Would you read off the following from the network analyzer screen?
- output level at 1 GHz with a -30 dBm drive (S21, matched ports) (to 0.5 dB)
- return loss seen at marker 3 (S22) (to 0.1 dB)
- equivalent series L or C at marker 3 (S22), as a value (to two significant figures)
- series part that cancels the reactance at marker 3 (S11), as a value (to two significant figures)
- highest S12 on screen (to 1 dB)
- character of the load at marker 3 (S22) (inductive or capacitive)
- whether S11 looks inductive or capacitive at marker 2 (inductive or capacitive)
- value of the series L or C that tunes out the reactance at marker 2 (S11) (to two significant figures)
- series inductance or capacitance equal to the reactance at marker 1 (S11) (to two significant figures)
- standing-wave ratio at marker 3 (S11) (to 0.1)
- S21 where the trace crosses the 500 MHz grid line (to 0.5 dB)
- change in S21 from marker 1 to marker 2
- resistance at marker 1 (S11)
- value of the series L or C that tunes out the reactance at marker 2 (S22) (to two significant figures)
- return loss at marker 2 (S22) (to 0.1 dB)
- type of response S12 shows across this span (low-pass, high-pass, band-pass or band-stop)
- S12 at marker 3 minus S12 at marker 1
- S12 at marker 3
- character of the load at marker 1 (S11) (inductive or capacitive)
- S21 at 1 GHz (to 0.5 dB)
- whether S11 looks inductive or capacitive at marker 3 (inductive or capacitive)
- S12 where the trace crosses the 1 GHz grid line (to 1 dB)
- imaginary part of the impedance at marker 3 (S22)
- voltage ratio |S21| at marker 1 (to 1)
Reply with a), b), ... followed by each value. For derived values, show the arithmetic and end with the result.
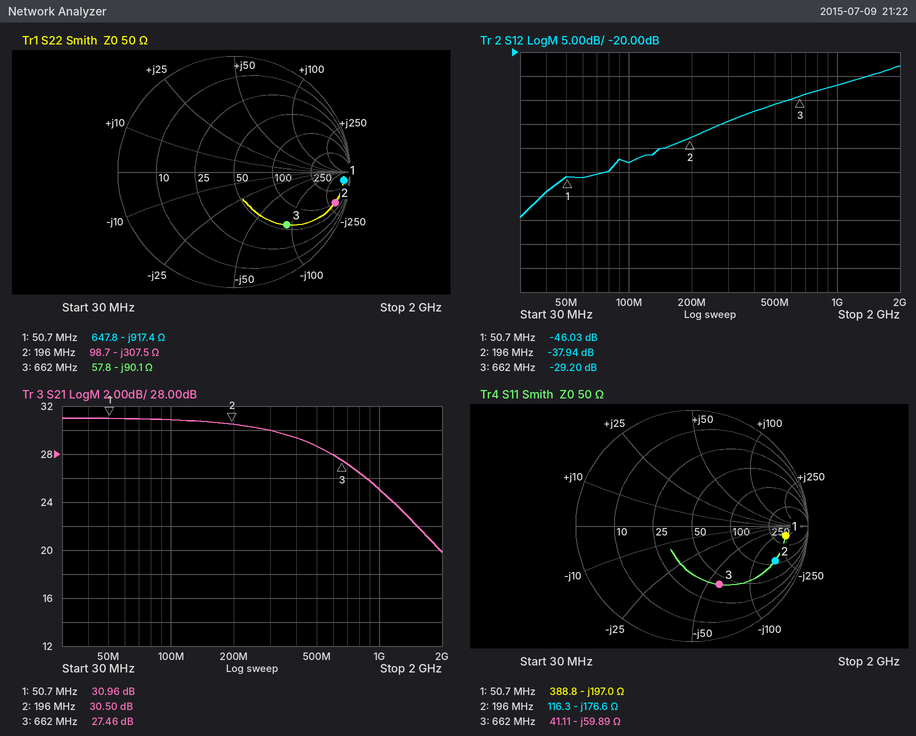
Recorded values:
a) -30 dBm + (25.0 dB) = -5.0 dBm
b) 3.8 dB
c) C = 1/(2π × 662 MHz × 90.1 Ω) ≈ 2.7 pF
d) L = 59.89 Ω/(2π × 662 MHz) ≈ 14 nH
e) -23 dB
f) capacitive
g) capacitive
h) L = 176.6 Ω/(2π × 196 MHz) ≈ 143 nH, so 140 nH to two significant figures
i) C = 1/(2π × 50.7 MHz × 197 Ω) ≈ 16 pF
j) 3.5
k) 28.5 dB
l) 30.5 − (30.96) = -0.46 dB
m) 388.8 Ω
n) L = 307.5 Ω/(2π × 196 MHz) ≈ 250 nH
o) 0.8 dB
p) high-pass
q) -29.2 − (-46.03) = 16.83 dB
r) -29.20 dB
s) capacitive
t) 25.0 dB
u) capacitive
v) -27 dB
w) -90.1 Ω
x) 10^(30.96/20) ≈ 35
